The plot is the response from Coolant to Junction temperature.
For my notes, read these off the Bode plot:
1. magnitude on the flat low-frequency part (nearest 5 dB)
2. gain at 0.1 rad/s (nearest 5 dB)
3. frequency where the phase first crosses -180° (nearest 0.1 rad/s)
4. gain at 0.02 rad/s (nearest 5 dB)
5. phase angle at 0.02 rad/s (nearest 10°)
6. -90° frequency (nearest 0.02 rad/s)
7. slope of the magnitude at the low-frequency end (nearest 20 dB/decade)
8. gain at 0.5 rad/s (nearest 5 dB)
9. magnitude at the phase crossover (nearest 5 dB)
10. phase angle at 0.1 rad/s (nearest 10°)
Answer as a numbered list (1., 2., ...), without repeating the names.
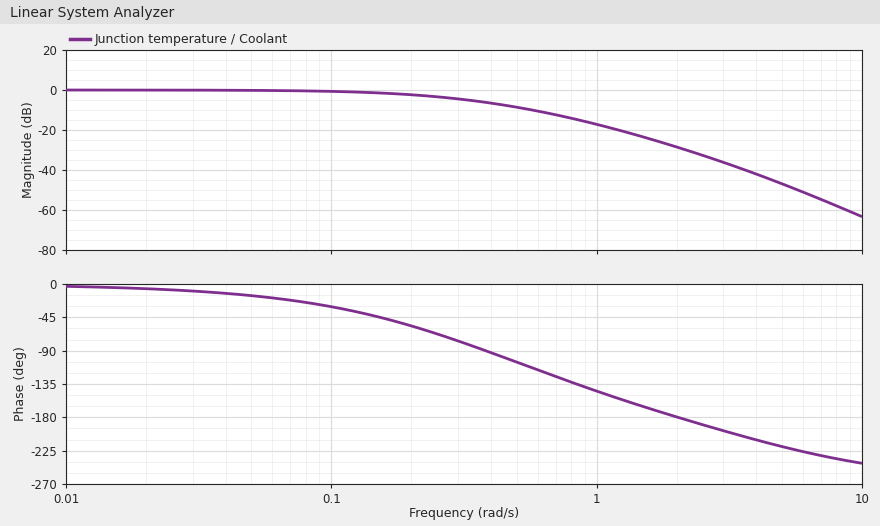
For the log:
1. 0 dB
2. 0 dB
3. 2.0 rad/s
4. 0 dB
5. -10°
6. 0.38 rad/s
7. 0 dB/decade
8. -10 dB
9. -30 dB
10. -30°
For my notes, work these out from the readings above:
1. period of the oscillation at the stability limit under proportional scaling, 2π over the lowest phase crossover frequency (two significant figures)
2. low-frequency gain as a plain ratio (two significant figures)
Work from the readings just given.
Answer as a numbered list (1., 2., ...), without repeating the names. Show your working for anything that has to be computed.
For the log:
1. 2π / 2 = 3.1 s
2. 10^(0 / 20) = 1.0
